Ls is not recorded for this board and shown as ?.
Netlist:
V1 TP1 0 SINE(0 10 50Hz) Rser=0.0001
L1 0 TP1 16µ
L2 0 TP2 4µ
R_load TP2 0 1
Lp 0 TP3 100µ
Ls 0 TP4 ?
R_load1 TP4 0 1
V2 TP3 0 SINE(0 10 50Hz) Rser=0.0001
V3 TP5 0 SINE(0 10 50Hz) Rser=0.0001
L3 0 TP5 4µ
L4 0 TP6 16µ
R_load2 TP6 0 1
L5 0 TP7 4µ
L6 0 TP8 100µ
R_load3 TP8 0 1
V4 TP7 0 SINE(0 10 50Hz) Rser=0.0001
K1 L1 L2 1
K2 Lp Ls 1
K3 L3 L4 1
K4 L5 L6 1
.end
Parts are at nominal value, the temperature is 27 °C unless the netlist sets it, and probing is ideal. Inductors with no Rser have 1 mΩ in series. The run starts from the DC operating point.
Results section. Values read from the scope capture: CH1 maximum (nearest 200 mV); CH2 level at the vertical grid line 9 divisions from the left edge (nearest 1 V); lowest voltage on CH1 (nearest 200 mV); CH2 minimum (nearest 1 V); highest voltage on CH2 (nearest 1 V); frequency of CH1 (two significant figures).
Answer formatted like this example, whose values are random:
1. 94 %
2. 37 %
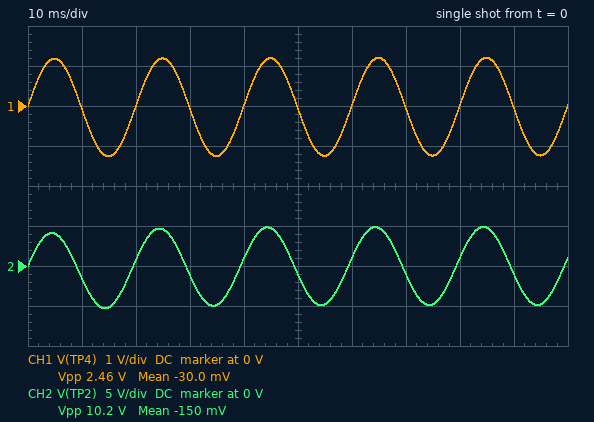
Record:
1. 1.2 V
2. -1 V
3. -1.2 V
4. -5 V
5. 5 V
6. 50 Hz
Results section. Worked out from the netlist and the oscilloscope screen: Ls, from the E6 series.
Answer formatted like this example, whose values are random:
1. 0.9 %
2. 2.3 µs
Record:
1. 1.5 µH
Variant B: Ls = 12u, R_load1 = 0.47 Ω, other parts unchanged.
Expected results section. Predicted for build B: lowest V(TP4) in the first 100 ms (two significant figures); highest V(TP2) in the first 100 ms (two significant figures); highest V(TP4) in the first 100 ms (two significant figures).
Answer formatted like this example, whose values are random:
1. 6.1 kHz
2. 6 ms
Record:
1. -3.6 V
2. 4.9 V
3. 3.4 V
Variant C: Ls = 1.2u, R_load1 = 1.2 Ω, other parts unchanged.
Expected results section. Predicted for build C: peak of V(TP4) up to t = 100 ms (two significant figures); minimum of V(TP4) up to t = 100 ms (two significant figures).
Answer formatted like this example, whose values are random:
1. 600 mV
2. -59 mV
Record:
1. 1.1 V
2. -1.1 V
